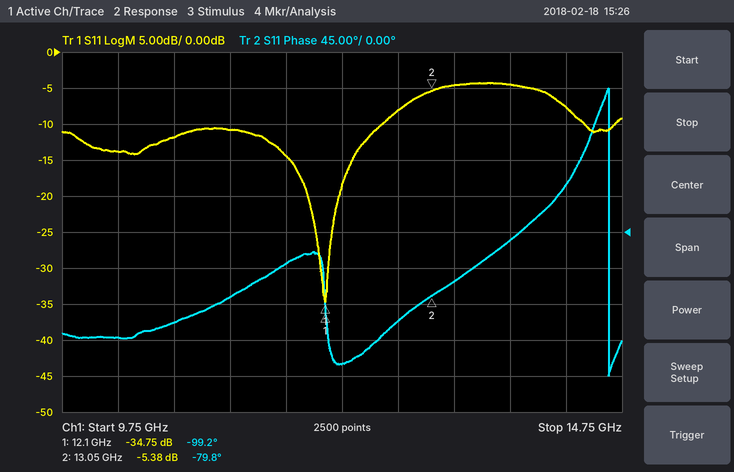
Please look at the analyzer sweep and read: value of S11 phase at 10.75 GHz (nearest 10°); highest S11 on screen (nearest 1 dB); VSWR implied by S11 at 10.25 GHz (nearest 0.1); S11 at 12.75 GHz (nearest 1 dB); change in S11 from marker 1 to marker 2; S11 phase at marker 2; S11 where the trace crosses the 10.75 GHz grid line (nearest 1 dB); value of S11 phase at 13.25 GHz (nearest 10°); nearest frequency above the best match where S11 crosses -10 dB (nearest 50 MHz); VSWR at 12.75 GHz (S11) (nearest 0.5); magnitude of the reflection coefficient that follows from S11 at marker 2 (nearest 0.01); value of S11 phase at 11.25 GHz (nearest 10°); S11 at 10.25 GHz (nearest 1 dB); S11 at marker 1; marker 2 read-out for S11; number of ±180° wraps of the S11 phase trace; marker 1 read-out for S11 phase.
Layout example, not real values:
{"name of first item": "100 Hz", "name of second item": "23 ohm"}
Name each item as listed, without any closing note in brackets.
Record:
{"value of S11 phase at 10.75 GHz": "-110°", "highest S11 on screen": "-4 dB", "VSWR implied by S11 at 10.25 GHz": "1.5", "S11 at 12.75 GHz": "-8 dB", "change in S11 from marker 1 to marker 2": "29.37 dB", "S11 phase at marker 2": "-79.8°", "S11 where the trace crosses the 10.75 GHz grid line": "-12 dB", "value of S11 phase at 13.25 GHz": "-60°", "nearest frequency above the best match where S11 crosses -10 dB": "12.60 GHz", "VSWR at 12.75 GHz (S11)": "2.5", "magnitude of the reflection coefficient that follows from S11 at marker 2": "0.54", "value of S11 phase at 11.25 GHz": "-80°", "S11 at 10.25 GHz": "-14 dB", "S11 at marker 1": "-34.75 dB", "marker 2 read-out for S11": "-5.38 dB", "number of ±180° wraps of the S11 phase trace": "1", "marker 1 read-out for S11 phase": "-99.2°"}
